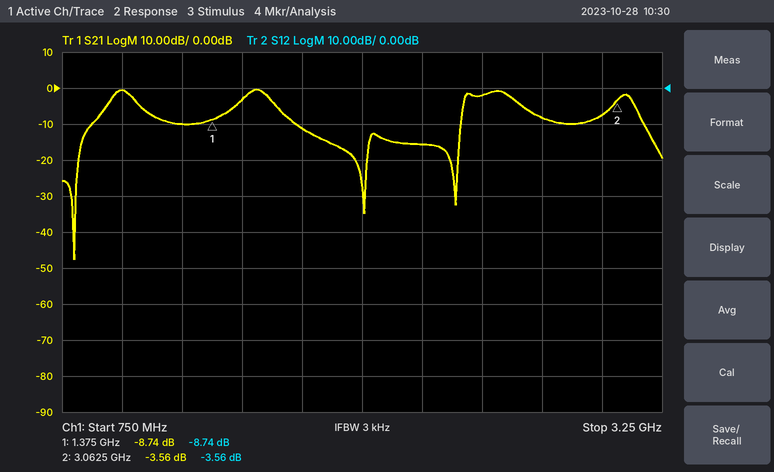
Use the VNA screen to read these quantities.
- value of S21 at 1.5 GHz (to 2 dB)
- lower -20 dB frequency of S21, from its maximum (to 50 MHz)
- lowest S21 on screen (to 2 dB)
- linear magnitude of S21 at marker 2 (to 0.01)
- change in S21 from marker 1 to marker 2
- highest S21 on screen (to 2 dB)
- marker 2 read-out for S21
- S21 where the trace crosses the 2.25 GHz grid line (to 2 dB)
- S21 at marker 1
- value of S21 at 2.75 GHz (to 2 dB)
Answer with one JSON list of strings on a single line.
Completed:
["-4 dB", "800 MHz", "-48 dB", "0.66", "5.18 dB", "0 dB", "-3.56 dB", "-16 dB", "-8.74 dB", "-8 dB"]
